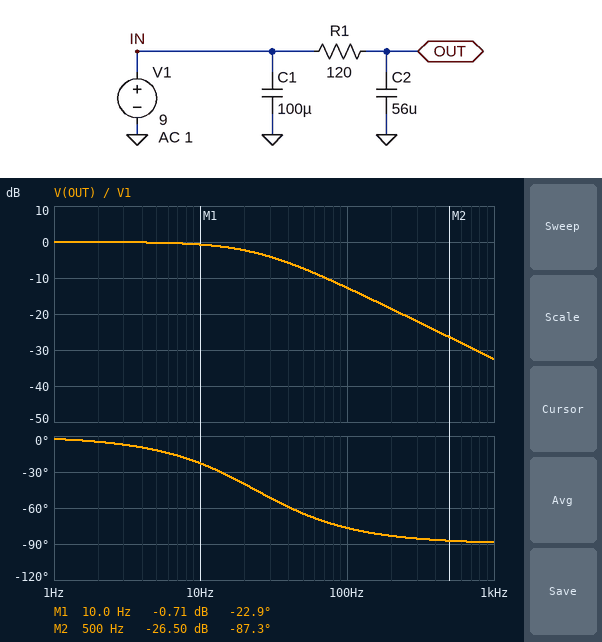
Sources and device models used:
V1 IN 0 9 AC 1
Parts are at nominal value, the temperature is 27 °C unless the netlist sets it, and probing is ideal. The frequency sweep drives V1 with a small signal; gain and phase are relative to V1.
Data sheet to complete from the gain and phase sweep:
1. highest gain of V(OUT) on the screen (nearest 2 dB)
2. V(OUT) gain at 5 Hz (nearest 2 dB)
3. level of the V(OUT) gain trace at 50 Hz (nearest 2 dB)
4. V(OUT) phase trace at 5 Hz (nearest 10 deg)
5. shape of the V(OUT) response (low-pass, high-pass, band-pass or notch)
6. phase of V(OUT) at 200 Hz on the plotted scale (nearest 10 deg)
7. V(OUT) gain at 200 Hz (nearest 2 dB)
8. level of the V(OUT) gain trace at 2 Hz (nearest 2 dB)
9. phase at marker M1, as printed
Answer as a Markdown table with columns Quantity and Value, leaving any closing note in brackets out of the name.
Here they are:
| Quantity | Value |
|---|---|
| highest gain of V(OUT) on the screen | 0 dB |
| V(OUT) gain at 5 Hz | 0 dB |
| level of the V(OUT) gain trace at 50 Hz | -8 dB |
| V(OUT) phase trace at 5 Hz | -10 deg |
| shape of the V(OUT) response | low-pass |
| phase of V(OUT) at 200 Hz on the plotted scale | -80 deg |
| V(OUT) gain at 200 Hz | -18 dB |
| level of the V(OUT) gain trace at 2 Hz | 0 dB |
| phase at marker M1, as printed | -22.9 deg |
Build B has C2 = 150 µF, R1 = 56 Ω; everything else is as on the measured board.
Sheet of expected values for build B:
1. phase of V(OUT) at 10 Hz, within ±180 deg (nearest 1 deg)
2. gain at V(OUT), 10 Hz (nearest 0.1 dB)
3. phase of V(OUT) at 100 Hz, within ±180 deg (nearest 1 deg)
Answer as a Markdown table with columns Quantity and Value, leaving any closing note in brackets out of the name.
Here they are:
| Quantity | Value |
|---|---|
| phase of V(OUT) at 10 Hz, within ±180 deg | -28 deg |
| gain at V(OUT), 10 Hz | -1.1 dB |
| phase of V(OUT) at 100 Hz, within ±180 deg | -79 deg |
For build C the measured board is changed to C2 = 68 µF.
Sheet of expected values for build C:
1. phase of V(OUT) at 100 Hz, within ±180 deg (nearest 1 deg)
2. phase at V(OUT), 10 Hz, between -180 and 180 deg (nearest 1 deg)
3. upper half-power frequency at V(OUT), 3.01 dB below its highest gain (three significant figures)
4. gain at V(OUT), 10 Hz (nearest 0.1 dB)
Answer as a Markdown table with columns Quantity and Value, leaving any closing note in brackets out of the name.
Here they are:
| Quantity | Value |
|---|---|
| phase of V(OUT) at 100 Hz, within ±180 deg | -79 deg |
| phase at V(OUT), 10 Hz, between -180 and 180 deg | -27 deg |
| upper half-power frequency at V(OUT), 3.01 dB below its highest gain | 19.5 Hz |
| gain at V(OUT), 10 Hz | -1.0 dB |
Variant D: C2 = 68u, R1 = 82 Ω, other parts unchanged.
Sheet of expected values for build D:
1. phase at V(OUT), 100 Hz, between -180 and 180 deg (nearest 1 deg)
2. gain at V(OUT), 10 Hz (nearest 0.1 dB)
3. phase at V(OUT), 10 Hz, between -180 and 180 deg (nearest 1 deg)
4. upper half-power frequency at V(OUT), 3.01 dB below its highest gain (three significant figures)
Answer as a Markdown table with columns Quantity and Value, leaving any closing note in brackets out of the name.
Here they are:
| Quantity | Value |
|---|---|
| phase at V(OUT), 100 Hz, between -180 and 180 deg | -74 deg |
| gain at V(OUT), 10 Hz | -0.5 dB |
| phase at V(OUT), 10 Hz, between -180 and 180 deg | -19 deg |
| upper half-power frequency at V(OUT), 3.01 dB below its highest gain | 28.5 Hz |
